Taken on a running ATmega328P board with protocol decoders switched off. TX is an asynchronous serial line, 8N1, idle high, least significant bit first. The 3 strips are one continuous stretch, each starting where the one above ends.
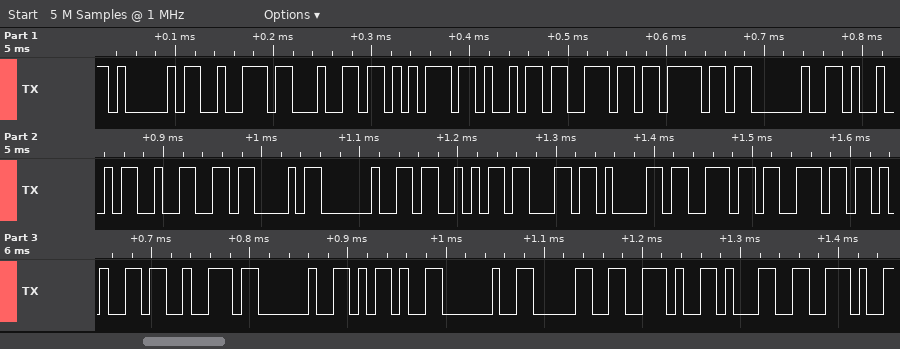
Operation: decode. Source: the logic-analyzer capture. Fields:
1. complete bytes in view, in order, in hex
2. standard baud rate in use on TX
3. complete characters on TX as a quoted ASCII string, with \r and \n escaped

41 72 64 75 69 6E 6F 20 49 32 43 20 53 63 61 6E 6E 65 72 20 2D 20 30 2E 31 2E
115200 baud
"Arduino I2C Scanner - 0.1."
